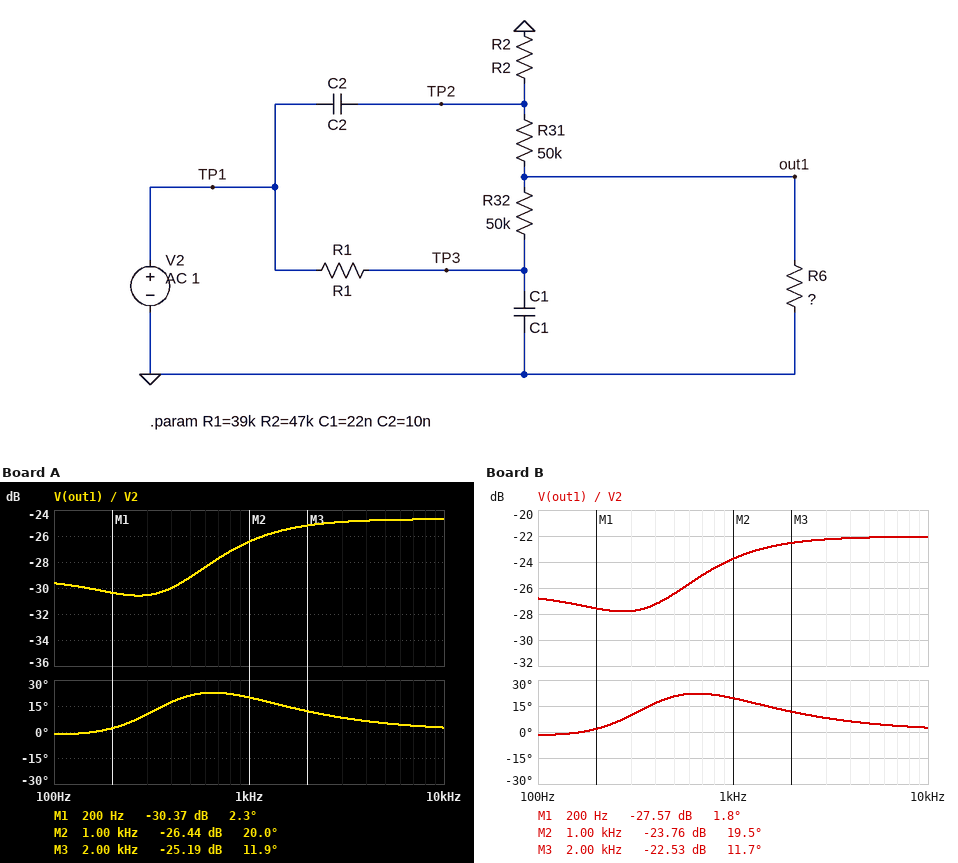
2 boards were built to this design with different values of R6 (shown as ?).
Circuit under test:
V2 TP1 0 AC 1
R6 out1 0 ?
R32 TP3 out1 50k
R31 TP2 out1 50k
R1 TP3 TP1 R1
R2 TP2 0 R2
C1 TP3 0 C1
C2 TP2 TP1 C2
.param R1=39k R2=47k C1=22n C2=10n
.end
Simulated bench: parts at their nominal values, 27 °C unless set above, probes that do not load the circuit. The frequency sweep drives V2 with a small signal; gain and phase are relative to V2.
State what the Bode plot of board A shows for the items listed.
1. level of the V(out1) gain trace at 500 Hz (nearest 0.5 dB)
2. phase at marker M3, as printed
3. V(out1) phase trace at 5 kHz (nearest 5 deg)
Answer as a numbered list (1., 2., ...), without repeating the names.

1. -29.0 dB
2. 11.9 deg
3. 5 deg
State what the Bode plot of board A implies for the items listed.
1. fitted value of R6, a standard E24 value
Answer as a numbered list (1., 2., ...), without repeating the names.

1. 3.3 kΩ
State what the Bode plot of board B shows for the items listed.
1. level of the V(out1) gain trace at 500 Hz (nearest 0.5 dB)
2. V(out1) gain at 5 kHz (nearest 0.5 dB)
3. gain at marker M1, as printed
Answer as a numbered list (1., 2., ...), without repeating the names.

1. -26.5 dB
2. -22.0 dB
3. -27.57 dB
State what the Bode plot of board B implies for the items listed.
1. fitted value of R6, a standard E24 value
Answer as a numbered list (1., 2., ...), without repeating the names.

1. 4.7 kΩ
